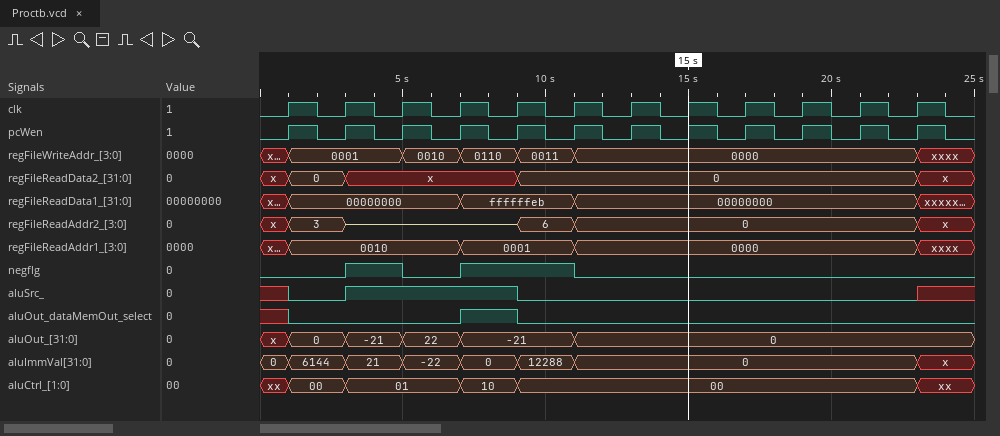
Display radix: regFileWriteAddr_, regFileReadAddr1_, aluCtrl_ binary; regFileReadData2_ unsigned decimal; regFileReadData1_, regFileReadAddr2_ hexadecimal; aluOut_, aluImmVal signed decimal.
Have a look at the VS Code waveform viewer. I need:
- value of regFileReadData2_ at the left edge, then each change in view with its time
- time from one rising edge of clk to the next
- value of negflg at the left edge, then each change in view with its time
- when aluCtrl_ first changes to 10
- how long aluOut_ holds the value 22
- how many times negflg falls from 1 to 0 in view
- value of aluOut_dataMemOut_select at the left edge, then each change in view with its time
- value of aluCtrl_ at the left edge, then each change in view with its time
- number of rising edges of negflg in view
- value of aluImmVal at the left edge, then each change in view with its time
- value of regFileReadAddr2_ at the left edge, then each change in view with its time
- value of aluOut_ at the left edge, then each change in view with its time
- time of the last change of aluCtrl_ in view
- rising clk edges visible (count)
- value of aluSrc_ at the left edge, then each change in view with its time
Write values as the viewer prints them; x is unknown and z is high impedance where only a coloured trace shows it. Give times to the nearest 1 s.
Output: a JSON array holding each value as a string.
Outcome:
["x, 0 at 1 s, x at 3 s, 0 at 9 s, x at 23 s", "2 s", "0, 1 at 3 s, 0 at 5 s, 1 at 7 s, 0 at 11 s", "7 s", "2 s", "2", "x, 0 at 1 s, 1 at 7 s, 0 at 9 s", "xx, 00 at 1 s, 01 at 3 s, 10 at 7 s, 00 at 9 s, xx at 23 s", "2", "0, 6144 at 1 s, 21 at 3 s, -22 at 5 s, 0 at 7 s, 12288 at 9 s, 0 at 11 s, x at 23 s", "x, 3 at 1 s, z at 3 s, 6 at 9 s, 0 at 11 s, x at 23 s", "x, 0 at 1 s, -21 at 3 s, 22 at 5 s, -21 at 7 s, 0 at 11 s", "23 s", "12", "x, 0 at 1 s, 1 at 3 s, 0 at 9 s, x at 23 s"]
